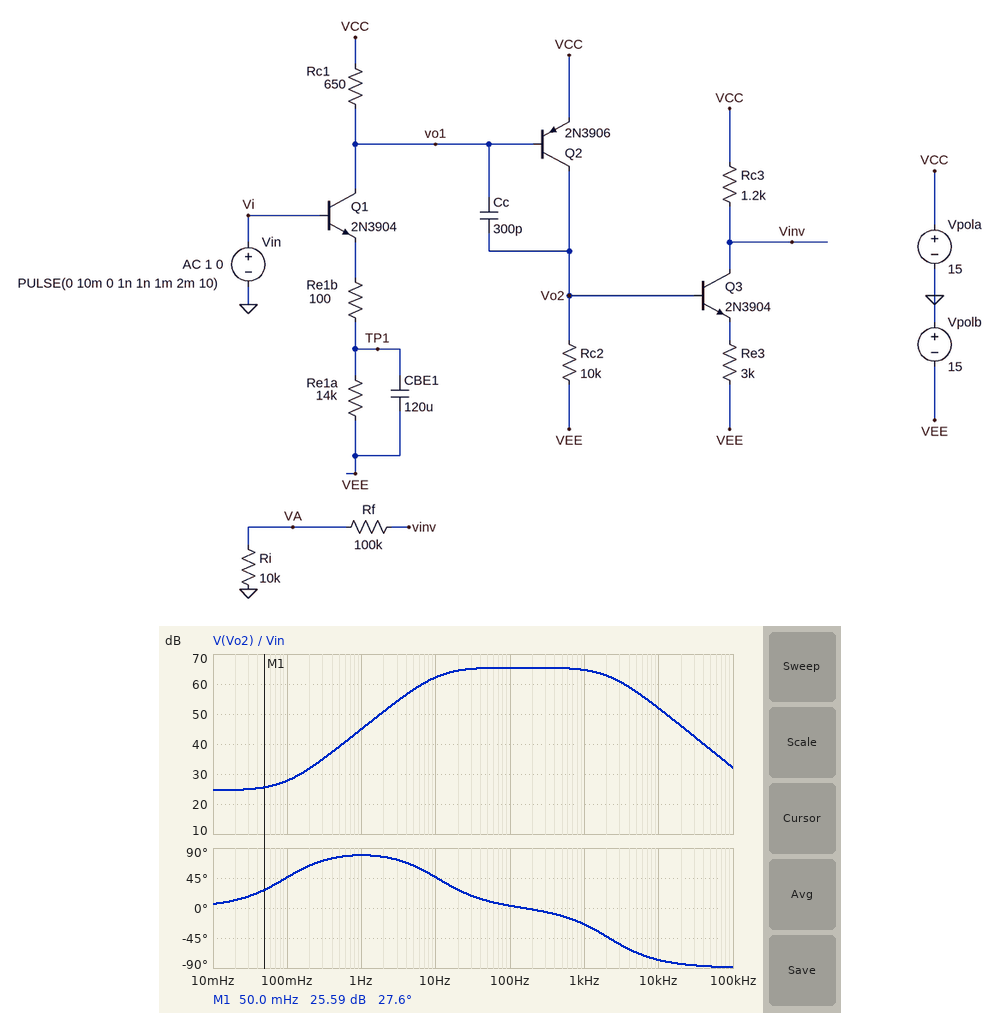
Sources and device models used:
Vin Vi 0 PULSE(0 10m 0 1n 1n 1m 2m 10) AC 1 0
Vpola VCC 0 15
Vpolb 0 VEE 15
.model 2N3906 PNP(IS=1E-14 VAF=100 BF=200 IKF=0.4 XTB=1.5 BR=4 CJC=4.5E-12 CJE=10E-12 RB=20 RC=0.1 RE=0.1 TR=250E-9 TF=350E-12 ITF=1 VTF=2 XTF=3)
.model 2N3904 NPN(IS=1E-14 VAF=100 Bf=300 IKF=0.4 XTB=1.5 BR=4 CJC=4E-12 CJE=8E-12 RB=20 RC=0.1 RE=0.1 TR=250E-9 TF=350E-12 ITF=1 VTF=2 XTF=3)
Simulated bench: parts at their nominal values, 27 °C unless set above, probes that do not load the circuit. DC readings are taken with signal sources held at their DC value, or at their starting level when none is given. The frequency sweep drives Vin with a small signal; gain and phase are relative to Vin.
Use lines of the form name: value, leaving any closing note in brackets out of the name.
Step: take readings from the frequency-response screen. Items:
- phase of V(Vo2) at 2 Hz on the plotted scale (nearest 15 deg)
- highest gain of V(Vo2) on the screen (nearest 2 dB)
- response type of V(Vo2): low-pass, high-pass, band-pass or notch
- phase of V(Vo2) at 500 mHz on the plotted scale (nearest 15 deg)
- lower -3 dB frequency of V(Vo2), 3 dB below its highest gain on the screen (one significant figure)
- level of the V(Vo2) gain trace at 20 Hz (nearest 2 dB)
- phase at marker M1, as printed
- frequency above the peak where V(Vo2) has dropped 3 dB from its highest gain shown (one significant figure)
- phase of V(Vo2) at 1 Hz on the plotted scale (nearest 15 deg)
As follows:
phase of V(Vo2) at 2 Hz on the plotted scale: 75 deg
highest gain of V(Vo2) on the screen: 66 dB
response type of V(Vo2): low-pass, high-pass, band-pass or notch: band-pass
phase of V(Vo2) at 500 mHz on the plotted scale: 75 deg
lower -3 dB frequency of V(Vo2), 3 dB below its highest gain on the screen: 10 Hz
level of the V(Vo2) gain trace at 20 Hz: 64 dB
phase at marker M1, as printed: 27.6 deg
frequency above the peak where V(Vo2) has dropped 3 dB from its highest gain shown: 2 kHz
phase of V(Vo2) at 1 Hz on the plotted scale: 75 deg
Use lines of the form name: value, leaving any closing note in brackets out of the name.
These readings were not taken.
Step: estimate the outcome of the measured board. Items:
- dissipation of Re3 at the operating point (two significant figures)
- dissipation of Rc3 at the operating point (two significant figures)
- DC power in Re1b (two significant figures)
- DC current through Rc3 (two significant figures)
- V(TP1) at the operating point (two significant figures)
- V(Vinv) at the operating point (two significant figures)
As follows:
dissipation of Re3 at the operating point: 42 mW
dissipation of Rc3 at the operating point: 18 mW
DC power in Re1b: 100 µW
DC current through Rc3: 3.8 mA
V(TP1) at the operating point: -750 mV
V(Vinv) at the operating point: 10 V
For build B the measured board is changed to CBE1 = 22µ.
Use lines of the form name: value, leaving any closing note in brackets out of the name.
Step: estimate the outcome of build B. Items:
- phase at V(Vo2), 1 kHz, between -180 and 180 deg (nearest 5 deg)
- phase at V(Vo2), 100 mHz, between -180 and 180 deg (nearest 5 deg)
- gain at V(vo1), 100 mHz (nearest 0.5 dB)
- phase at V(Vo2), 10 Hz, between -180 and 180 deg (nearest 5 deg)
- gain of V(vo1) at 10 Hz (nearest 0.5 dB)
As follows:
phase at V(Vo2), 1 kHz, between -180 and 180 deg: -20 deg
phase at V(Vo2), 100 mHz, between -180 and 180 deg: 10 deg
gain at V(vo1), 100 mHz: -27.5 dB
phase at V(Vo2), 10 Hz, between -180 and 180 deg: 75 deg
gain of V(vo1) at 10 Hz: -2.0 dB
